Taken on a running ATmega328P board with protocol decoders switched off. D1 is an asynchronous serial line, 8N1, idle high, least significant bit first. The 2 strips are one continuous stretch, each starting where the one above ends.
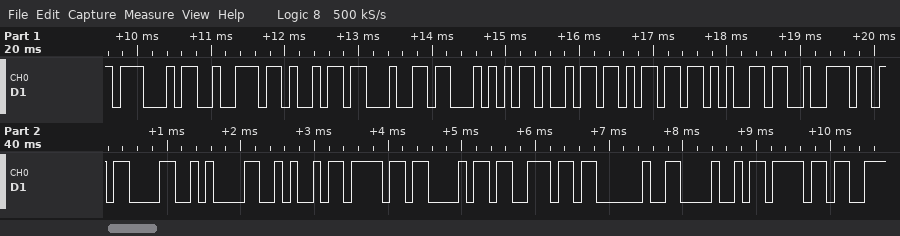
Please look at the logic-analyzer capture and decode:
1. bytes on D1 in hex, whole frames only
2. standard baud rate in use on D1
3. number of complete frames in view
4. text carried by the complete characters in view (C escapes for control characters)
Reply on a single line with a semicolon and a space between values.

47 72 69 64 54 69 6D 65 72 0D 0A 4A 6F 68 6E 20 48 6F; 9600 baud; 18; "GridTimer\r\nJohn Ho"
